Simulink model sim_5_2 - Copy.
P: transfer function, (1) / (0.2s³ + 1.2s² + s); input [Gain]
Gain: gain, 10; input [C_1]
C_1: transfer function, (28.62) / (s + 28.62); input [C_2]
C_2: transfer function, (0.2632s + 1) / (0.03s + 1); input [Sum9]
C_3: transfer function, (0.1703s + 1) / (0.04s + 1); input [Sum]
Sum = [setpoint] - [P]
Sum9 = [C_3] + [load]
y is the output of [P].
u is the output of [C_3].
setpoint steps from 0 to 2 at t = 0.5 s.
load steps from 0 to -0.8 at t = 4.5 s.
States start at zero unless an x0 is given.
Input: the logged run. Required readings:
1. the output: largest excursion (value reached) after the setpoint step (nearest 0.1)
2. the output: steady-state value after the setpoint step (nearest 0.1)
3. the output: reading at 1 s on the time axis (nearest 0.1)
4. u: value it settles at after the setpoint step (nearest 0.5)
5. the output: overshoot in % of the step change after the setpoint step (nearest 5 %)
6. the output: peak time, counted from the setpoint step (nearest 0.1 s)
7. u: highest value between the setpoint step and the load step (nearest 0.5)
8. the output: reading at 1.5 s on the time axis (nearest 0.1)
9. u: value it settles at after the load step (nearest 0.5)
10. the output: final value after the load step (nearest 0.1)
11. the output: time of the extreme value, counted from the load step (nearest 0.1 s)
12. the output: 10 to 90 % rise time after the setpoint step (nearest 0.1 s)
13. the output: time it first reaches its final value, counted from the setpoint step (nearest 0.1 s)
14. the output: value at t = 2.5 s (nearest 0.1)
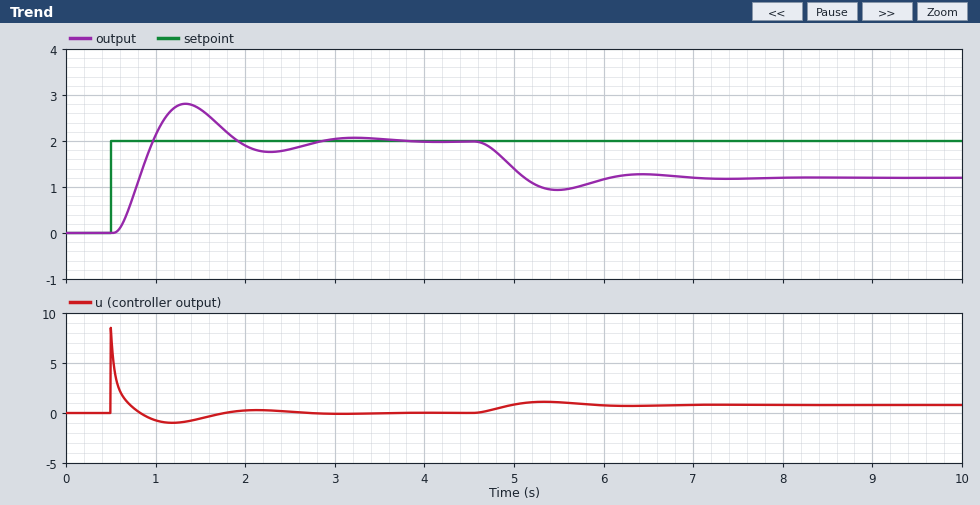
2.8
2.0
2.1
0.0
40 %
0.8 s
8.5
2.7
1.0
1.2
1.0 s
0.3 s
0.5 s
1.8
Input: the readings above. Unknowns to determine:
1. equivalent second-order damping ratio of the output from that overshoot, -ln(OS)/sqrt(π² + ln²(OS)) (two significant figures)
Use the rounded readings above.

0.28
